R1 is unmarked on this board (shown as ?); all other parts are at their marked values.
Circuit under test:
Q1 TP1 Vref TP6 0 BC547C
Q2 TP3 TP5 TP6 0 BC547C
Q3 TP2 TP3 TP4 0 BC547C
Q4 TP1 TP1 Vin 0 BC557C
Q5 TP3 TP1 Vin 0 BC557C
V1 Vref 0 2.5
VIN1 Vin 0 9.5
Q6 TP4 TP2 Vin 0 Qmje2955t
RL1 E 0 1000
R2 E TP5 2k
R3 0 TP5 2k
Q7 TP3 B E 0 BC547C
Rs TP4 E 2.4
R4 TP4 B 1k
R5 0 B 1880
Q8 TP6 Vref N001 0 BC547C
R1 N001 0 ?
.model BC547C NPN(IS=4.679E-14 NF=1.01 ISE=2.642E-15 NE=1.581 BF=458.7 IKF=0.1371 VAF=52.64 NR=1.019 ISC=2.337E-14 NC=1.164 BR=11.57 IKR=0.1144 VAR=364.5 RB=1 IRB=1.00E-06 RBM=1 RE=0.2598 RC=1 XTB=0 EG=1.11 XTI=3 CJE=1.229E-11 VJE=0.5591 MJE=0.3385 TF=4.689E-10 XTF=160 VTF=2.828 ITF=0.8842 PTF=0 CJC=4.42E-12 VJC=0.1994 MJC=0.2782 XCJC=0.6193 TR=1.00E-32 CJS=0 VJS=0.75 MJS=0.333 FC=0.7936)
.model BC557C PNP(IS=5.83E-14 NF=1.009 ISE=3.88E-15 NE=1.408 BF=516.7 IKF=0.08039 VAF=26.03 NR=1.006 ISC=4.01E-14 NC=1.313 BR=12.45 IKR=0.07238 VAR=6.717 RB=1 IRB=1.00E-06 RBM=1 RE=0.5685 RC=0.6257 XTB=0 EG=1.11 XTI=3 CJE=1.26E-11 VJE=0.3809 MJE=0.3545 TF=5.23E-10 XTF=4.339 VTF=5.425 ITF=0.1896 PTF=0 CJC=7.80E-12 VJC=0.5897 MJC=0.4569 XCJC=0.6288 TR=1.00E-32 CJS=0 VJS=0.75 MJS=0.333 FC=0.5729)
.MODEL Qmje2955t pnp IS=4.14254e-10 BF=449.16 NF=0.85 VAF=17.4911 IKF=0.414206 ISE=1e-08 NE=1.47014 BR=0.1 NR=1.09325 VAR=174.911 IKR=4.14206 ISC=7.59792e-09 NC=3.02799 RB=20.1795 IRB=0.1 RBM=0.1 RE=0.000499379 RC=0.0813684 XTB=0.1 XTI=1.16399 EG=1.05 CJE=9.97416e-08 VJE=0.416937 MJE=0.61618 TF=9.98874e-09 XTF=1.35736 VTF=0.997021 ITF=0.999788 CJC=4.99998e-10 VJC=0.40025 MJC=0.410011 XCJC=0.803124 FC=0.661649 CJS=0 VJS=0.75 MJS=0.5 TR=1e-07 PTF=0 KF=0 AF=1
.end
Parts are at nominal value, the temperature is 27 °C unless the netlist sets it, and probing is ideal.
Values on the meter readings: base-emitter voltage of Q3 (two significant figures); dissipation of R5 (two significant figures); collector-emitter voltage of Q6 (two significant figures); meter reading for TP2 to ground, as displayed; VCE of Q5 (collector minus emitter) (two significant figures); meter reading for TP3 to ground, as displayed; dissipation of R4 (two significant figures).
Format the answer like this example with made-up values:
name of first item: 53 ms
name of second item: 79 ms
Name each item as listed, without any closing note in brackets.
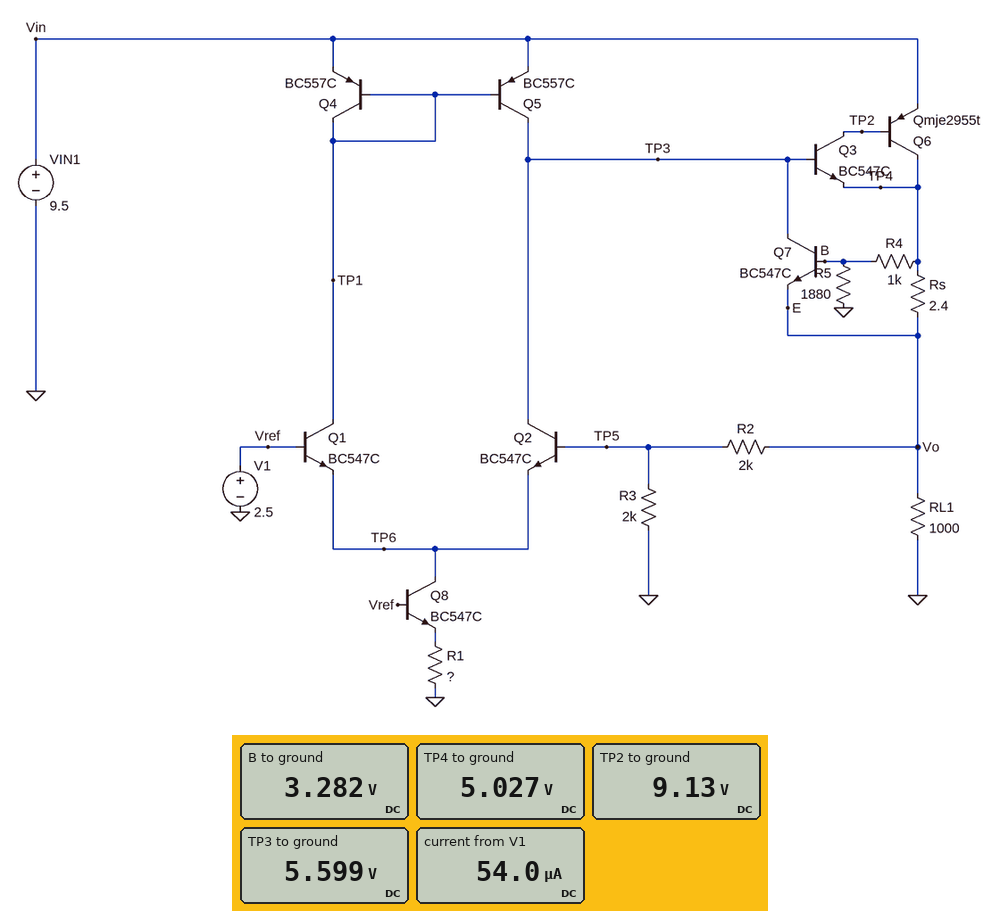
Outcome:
base-emitter voltage of Q3: 570 mV
dissipation of R5: 5.7 mW
collector-emitter voltage of Q6: -4.5 V
meter reading for TP2 to ground, as displayed: 9.13 V
VCE of Q5 (collector minus emitter): -3.9 V
meter reading for TP3 to ground, as displayed: 5.599 V
dissipation of R4: 3.0 mW
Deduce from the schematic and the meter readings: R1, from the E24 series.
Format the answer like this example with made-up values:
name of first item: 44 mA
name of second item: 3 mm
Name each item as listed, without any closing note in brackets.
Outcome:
R1, from the E24 series: 1.5 kΩ
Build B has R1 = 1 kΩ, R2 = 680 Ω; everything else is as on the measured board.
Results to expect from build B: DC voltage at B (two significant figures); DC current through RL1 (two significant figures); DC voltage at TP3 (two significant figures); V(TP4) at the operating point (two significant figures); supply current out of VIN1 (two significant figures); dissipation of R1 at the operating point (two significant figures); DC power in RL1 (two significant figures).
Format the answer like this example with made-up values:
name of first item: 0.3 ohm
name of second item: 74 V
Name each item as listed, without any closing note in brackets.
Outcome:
DC voltage at B: 2.2 V
DC current through RL1: 3.4 mA
DC voltage at TP3: 3.9 V
V(TP4) at the operating point: 3.4 V
supply current out of VIN1: 7.6 mA
dissipation of R1 at the operating point: 3.4 mW
DC power in RL1: 11 mW
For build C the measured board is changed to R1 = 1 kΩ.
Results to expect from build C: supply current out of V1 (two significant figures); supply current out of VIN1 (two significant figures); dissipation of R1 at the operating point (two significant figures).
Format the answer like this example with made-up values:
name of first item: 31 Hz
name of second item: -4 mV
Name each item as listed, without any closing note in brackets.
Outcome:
supply current out of V1: 81 µA
supply current out of VIN1: 9.8 mA
dissipation of R1 at the operating point: 3.4 mW
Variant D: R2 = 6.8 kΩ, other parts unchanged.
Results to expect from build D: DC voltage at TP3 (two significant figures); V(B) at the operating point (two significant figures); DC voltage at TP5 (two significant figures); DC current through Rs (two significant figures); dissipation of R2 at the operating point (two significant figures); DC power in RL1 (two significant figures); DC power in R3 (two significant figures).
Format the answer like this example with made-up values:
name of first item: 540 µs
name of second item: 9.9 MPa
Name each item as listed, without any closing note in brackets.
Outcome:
DC voltage at TP3: 9.5 V
V(B) at the operating point: 5.8 V
DC voltage at TP5: 2.0 V
DC current through Rs: 9.9 mA
dissipation of R2 at the operating point: 6.9 mW
DC power in RL1: 79 mW
DC power in R3: 2.0 mW
